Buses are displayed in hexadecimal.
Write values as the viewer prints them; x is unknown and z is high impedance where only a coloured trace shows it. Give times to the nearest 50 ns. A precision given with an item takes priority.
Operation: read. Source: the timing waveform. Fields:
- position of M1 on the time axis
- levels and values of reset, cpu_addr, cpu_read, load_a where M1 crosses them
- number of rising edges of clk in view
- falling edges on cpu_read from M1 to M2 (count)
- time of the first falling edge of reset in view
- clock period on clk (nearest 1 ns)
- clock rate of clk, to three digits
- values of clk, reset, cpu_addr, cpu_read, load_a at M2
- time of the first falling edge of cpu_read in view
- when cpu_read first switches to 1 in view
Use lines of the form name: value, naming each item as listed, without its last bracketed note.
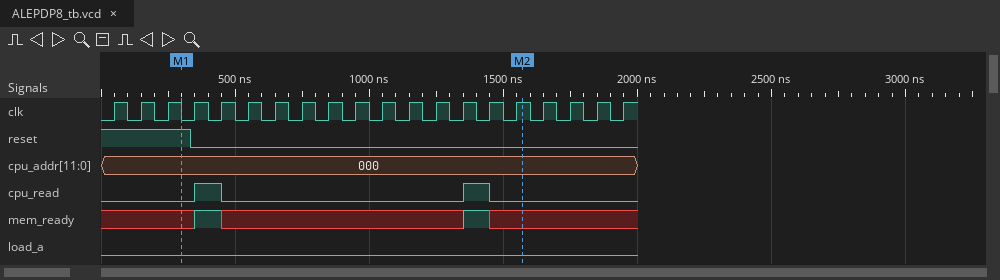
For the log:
position of M1 on the time axis: 300 ns
levels and values of reset, cpu_addr, cpu_read, load_a where M1 crosses them: reset=1, cpu_addr=000, cpu_read=0, load_a=0
number of rising edges of clk in view: 20
falling edges on cpu_read from M1 to M2: 2
time of the first falling edge of reset in view: 350 ns
clock period on clk: 100 ns
clock rate of clk, to three digits: 10.0 MHz
values of clk, reset, cpu_addr, cpu_read, load_a at M2: clk=1, reset=0, cpu_addr=000, cpu_read=0, load_a=0
time of the first falling edge of cpu_read in view: 450 ns
when cpu_read first switches to 1 in view: 350 ns
